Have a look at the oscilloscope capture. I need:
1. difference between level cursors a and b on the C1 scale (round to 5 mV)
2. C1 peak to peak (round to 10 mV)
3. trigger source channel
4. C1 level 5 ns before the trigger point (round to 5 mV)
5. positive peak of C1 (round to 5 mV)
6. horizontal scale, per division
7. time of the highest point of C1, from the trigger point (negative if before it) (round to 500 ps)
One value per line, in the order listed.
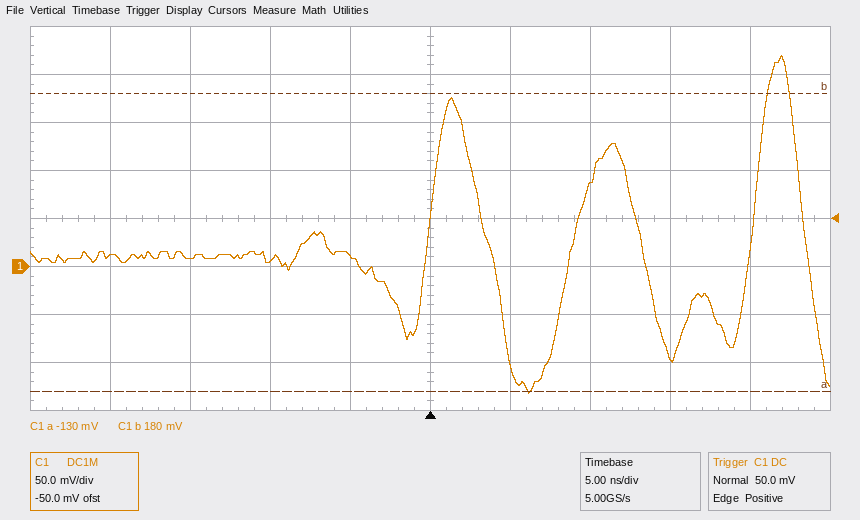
310 mV
350 mV
C1
10 mV
220 mV
5 ns
+22.0 ns
